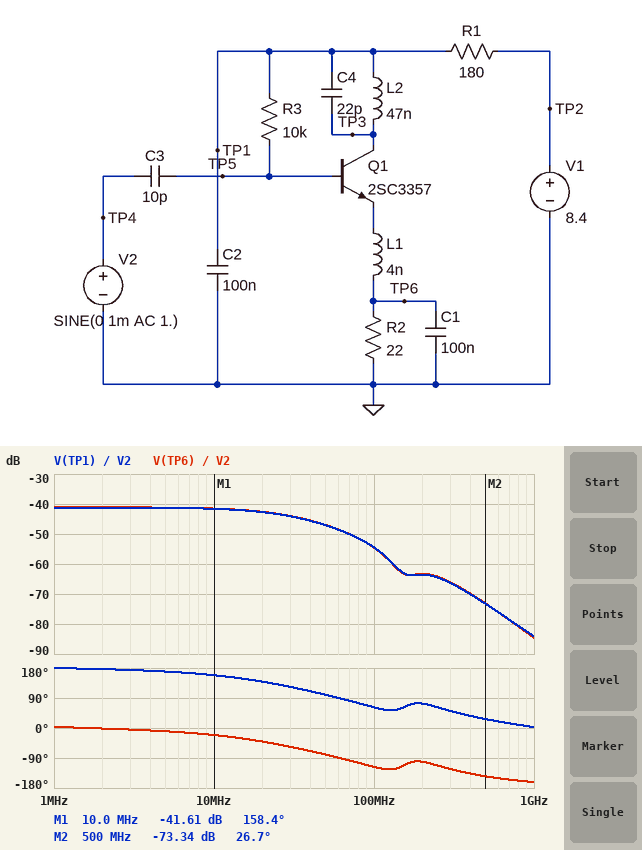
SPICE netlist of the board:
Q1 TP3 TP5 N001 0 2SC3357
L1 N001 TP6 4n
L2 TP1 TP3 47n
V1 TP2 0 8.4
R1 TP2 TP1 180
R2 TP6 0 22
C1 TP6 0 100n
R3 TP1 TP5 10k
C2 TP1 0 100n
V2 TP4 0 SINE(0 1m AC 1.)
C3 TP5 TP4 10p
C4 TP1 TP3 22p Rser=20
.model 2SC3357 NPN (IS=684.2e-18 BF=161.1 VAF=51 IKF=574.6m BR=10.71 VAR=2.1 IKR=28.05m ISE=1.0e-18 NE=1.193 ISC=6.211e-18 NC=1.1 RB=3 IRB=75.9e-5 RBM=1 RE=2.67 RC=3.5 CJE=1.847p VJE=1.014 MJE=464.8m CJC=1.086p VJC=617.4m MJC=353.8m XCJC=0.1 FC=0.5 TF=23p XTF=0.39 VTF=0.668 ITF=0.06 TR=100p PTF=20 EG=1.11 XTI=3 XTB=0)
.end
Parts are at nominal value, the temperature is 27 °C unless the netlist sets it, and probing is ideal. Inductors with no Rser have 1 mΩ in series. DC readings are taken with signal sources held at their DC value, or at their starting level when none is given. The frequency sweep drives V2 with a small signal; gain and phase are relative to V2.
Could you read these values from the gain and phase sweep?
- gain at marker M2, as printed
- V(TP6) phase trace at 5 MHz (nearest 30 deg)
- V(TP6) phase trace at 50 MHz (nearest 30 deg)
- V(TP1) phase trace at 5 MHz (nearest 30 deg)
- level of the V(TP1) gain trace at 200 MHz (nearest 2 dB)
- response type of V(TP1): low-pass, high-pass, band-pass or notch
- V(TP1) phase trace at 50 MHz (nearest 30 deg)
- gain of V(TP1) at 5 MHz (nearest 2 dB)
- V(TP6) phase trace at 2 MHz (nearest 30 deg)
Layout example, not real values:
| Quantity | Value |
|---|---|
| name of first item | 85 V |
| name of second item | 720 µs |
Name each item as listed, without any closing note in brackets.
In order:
| Quantity | Value |
|---|---|
| gain at marker M2, as printed | -73.34 dB |
| V(TP6) phase trace at 5 MHz | 0 deg |
| V(TP6) phase trace at 50 MHz | -90 deg |
| V(TP1) phase trace at 5 MHz | 180 deg |
| level of the V(TP1) gain trace at 200 MHz | -64 dB |
| response type of V(TP1): low-pass, high-pass, band-pass or notch | low-pass |
| V(TP1) phase trace at 50 MHz | 90 deg |
| gain of V(TP1) at 5 MHz | -42 dB |
| V(TP6) phase trace at 2 MHz | 0 deg |
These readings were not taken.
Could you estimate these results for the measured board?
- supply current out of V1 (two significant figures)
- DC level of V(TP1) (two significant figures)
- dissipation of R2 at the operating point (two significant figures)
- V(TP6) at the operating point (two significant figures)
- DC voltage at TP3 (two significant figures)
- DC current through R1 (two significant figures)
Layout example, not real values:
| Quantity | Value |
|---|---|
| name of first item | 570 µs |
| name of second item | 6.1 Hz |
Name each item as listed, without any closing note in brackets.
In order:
| Quantity | Value |
|---|---|
| supply current out of V1 | 25 mA |
| DC level of V(TP1) | 3.9 V |
| dissipation of R2 at the operating point | 14 mW |
| V(TP6) at the operating point | 550 mV |
| DC voltage at TP3 | 3.9 V |
| DC current through R1 | 25 mA |
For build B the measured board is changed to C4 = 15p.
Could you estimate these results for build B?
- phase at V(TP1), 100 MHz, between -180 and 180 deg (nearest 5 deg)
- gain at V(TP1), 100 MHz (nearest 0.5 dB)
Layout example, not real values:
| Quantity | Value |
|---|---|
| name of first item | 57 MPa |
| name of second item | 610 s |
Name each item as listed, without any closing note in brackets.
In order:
| Quantity | Value |
|---|---|
| phase at V(TP1), 100 MHz, between -180 and 180 deg | 65 deg |
| gain at V(TP1), 100 MHz | -54.0 dB |
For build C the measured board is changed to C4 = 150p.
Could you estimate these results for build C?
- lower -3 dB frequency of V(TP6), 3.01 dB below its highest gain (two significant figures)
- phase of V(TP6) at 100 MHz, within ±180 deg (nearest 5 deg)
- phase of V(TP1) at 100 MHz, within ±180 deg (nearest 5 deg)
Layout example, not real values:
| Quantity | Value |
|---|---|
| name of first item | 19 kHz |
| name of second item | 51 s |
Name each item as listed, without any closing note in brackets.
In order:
| Quantity | Value |
|---|---|
| lower -3 dB frequency of V(TP6), 3.01 dB below its highest gain | 93 kHz |
| phase of V(TP6) at 100 MHz, within ±180 deg | -100 deg |
| phase of V(TP1) at 100 MHz, within ±180 deg | 80 deg |
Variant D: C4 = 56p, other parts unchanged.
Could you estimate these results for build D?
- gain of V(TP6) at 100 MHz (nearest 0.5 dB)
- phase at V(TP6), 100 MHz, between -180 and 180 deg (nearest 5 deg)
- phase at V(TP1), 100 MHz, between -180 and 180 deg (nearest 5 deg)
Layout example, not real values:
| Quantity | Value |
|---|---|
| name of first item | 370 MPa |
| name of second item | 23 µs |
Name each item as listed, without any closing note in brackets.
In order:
| Quantity | Value |
|---|---|
| gain of V(TP6) at 100 MHz | -56.0 dB |
| phase at V(TP6), 100 MHz, between -180 and 180 deg | -105 deg |
| phase at V(TP1), 100 MHz, between -180 and 180 deg | 75 deg |
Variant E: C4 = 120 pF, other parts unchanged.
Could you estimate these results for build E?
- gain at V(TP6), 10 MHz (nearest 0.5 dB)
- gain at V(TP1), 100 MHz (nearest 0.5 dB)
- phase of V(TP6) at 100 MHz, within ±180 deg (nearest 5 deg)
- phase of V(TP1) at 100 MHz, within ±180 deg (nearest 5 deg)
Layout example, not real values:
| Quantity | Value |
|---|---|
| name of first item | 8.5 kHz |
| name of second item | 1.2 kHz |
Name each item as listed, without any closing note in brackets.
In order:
| Quantity | Value |
|---|---|
| gain at V(TP6), 10 MHz | -41.5 dB |
| gain at V(TP1), 100 MHz | -55.0 dB |
| phase of V(TP6) at 100 MHz, within ±180 deg | -100 deg |
| phase of V(TP1) at 100 MHz, within ±180 deg | 80 deg |
